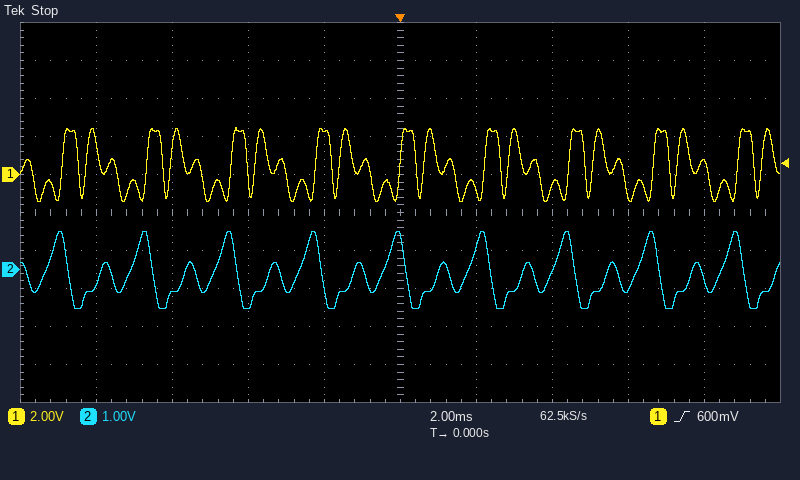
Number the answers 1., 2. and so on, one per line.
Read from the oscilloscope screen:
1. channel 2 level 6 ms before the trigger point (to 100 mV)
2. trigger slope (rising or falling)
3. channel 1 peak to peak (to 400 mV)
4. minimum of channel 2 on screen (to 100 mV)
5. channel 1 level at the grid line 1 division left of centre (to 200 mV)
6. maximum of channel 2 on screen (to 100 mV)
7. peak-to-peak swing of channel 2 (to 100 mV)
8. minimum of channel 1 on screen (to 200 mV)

1. -700 mV
2. rising
3. 4.0 V
4. -1.0 V
5. 2.4 V
6. 1.0 V
7. 2.0 V
8. -1.4 V
